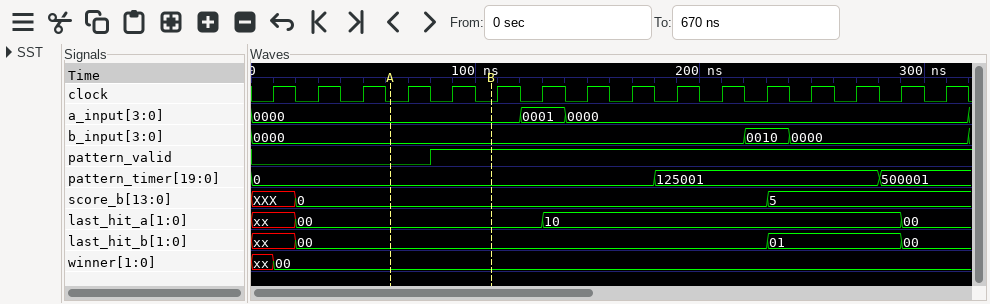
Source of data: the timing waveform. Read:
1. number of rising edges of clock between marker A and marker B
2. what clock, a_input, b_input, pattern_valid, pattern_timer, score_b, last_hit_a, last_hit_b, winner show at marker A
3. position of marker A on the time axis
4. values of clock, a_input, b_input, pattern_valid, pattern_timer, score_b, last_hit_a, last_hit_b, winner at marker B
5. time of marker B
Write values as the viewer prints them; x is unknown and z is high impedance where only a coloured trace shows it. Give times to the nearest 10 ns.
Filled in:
2
clock=0, a_input=0000, b_input=0000, pattern_valid=0, pattern_timer=0, score_b=0, last_hit_a=00, last_hit_b=00, winner=00
60 ns
clock=0, a_input=0000, b_input=0000, pattern_valid=1, pattern_timer=0, score_b=0, last_hit_a=00, last_hit_b=00, winner=00
110 ns
